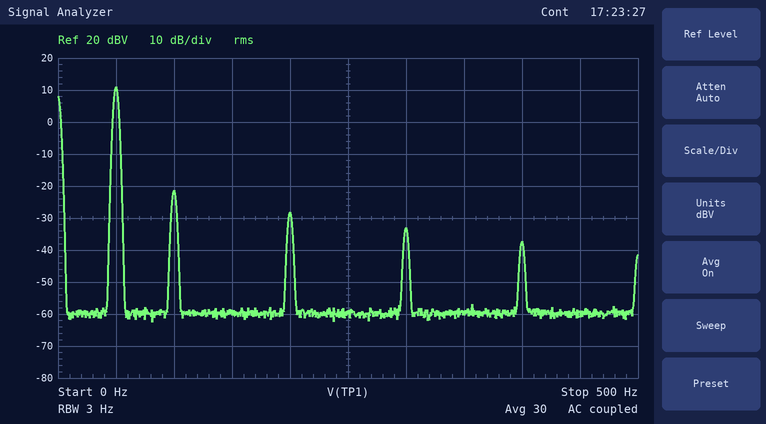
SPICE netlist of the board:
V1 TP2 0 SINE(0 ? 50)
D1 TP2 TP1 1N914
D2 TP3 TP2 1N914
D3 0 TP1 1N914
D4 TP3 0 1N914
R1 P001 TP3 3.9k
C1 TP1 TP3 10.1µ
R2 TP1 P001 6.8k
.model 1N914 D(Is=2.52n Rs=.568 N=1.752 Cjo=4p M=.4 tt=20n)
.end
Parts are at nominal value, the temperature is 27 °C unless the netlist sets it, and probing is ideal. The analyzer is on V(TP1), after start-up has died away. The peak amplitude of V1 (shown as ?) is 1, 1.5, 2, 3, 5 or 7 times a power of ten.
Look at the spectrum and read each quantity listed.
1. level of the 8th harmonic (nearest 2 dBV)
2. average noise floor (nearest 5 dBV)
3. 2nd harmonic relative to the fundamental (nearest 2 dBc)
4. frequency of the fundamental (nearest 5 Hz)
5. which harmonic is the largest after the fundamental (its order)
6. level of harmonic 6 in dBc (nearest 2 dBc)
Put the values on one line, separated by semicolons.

-38 dBV; -60 dBV; -32 dBc; 50 Hz; 2; -44 dBc
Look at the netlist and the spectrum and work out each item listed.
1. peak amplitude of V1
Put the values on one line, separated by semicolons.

10 V
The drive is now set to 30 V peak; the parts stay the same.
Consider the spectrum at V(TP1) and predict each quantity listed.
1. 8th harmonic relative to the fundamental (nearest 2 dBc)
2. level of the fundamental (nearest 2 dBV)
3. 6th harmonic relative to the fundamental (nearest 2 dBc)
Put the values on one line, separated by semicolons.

-46 dBc; 20 dBV; -42 dBc
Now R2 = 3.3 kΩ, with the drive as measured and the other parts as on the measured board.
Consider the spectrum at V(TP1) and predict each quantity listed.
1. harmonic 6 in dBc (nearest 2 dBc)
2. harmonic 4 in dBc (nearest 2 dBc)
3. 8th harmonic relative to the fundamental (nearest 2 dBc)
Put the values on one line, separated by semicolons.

-42 dBc; -36 dBc; -46 dBc
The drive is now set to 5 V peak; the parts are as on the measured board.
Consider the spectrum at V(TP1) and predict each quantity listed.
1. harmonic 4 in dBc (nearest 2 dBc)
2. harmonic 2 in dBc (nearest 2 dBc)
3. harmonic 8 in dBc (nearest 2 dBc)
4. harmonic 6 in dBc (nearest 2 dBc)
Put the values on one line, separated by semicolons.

-40 dBc; -34 dBc; -52 dBc; -46 dBc
